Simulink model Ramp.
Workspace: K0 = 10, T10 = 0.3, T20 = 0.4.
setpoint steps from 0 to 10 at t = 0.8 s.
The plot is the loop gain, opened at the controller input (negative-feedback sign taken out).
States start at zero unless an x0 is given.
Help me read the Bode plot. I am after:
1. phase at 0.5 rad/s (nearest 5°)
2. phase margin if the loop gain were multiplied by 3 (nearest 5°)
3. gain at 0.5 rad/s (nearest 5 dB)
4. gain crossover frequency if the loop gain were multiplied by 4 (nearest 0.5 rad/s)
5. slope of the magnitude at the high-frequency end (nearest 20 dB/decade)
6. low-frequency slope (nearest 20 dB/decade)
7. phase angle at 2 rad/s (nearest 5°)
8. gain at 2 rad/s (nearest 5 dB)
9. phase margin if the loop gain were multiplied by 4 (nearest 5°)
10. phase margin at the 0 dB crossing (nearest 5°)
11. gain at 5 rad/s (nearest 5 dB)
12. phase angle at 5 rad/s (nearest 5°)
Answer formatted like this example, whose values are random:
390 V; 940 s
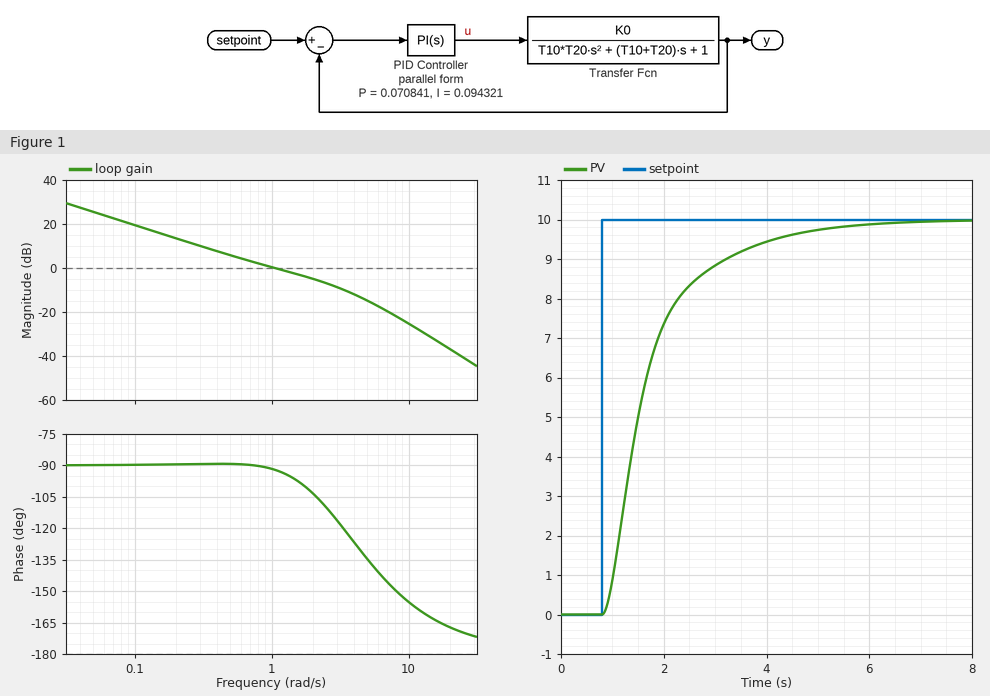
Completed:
-90°; 60°; 5 dB; 4.0 rad/s; -40 dB/decade; -20 dB/decade; -105°; -5 dB; 55°; 90°; -15 dB; -135°
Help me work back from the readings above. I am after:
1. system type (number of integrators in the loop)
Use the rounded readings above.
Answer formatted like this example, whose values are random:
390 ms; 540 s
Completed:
1
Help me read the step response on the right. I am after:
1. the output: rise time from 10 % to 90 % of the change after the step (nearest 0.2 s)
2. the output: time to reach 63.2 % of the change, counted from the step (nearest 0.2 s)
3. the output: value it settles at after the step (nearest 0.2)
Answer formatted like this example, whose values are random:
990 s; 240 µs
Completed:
2.2 s; 1.0 s; 10.0
